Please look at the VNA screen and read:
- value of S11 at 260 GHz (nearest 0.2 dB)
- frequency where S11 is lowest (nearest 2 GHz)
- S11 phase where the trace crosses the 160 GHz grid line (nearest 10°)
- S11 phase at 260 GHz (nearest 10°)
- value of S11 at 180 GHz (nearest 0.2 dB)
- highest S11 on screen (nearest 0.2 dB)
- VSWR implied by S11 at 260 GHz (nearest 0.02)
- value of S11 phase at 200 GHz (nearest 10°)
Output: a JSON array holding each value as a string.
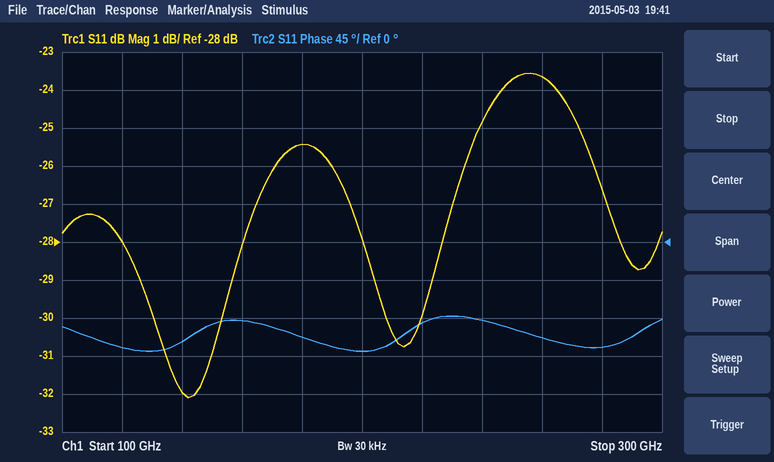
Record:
["-23.6 dB", "142 GHz", "-90°", "-110°", "-25.4 dB", "-23.6 dB", "1.14", "-130°"]
